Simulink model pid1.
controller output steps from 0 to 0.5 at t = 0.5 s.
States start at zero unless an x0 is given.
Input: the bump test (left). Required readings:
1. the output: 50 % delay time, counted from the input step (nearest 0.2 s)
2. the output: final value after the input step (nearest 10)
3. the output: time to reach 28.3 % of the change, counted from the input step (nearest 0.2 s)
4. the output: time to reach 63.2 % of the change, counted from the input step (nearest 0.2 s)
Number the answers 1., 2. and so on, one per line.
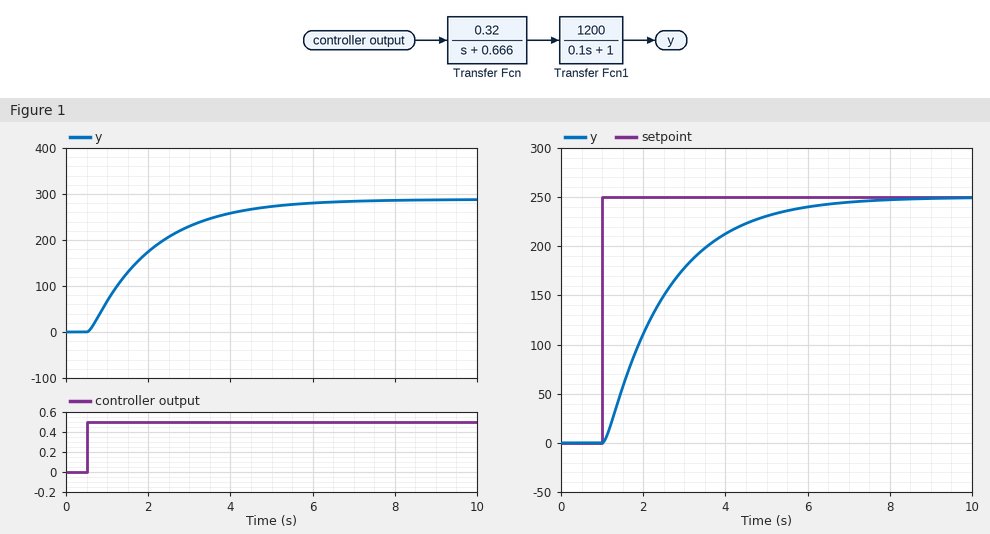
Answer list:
1. 1.2 s
2. 290
3. 0.6 s
4. 1.6 s
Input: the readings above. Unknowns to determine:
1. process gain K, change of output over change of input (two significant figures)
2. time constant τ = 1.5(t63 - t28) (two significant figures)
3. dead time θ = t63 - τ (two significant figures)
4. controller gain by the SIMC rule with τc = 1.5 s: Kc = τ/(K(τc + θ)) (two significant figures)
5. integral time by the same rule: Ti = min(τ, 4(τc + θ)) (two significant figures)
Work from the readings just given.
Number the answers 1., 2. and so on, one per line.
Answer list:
1. 580
2. 1.5 s
3. 0.10 s
4. 0.0016
5. 1.5 s
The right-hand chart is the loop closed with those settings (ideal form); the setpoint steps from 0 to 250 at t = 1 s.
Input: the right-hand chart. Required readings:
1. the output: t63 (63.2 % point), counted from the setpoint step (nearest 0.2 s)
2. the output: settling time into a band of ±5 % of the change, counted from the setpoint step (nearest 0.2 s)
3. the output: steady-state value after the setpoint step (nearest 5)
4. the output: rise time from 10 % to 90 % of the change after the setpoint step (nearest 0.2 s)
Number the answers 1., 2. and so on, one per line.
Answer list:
1. 1.6 s
2. 4.6 s
3. 250
4. 3.4 s
